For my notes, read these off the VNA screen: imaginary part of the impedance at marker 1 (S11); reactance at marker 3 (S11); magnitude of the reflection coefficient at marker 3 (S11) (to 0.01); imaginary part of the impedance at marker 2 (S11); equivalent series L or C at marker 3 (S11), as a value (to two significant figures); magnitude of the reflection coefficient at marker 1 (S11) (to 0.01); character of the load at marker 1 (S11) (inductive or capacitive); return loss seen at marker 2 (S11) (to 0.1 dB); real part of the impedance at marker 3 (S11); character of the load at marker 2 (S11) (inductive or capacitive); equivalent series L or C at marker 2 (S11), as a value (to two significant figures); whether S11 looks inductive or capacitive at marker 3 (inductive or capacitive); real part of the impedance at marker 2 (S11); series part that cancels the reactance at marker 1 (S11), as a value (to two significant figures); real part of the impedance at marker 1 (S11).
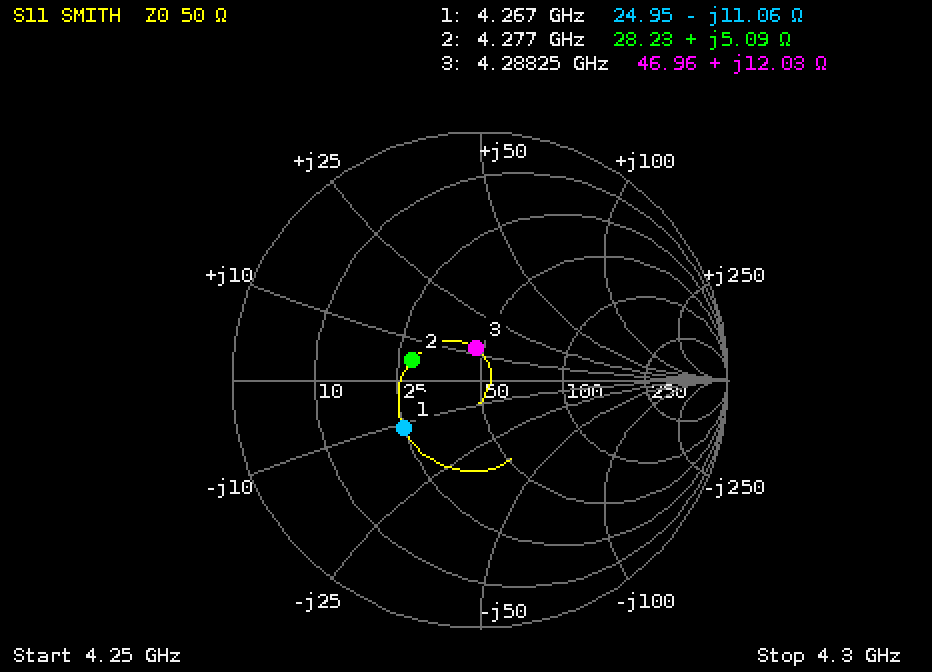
-11.06 Ω
+12.03 Ω
0.13
+5.09 Ω
450 pH
0.36
capacitive
10.9 dB
46.96 Ω
inductive
190 pH
inductive
28.23 Ω
410 pH
24.95 Ω
